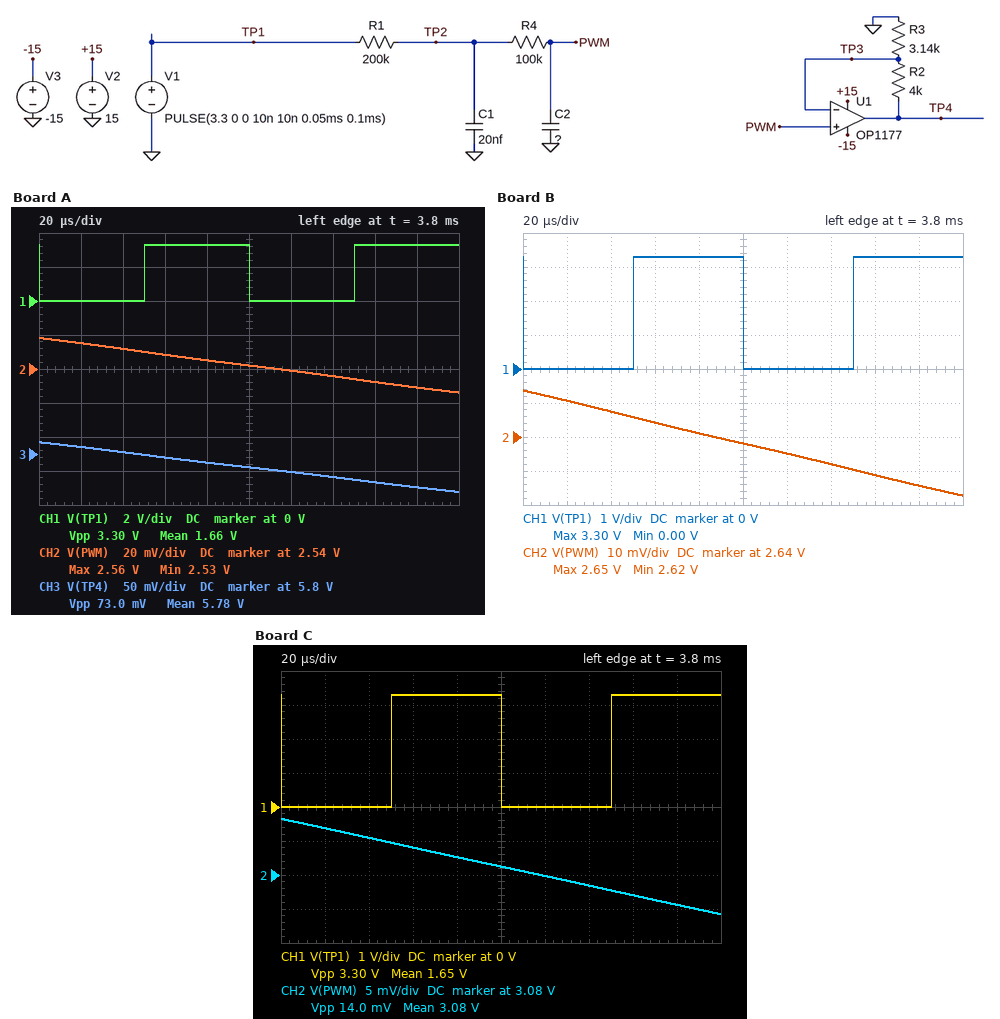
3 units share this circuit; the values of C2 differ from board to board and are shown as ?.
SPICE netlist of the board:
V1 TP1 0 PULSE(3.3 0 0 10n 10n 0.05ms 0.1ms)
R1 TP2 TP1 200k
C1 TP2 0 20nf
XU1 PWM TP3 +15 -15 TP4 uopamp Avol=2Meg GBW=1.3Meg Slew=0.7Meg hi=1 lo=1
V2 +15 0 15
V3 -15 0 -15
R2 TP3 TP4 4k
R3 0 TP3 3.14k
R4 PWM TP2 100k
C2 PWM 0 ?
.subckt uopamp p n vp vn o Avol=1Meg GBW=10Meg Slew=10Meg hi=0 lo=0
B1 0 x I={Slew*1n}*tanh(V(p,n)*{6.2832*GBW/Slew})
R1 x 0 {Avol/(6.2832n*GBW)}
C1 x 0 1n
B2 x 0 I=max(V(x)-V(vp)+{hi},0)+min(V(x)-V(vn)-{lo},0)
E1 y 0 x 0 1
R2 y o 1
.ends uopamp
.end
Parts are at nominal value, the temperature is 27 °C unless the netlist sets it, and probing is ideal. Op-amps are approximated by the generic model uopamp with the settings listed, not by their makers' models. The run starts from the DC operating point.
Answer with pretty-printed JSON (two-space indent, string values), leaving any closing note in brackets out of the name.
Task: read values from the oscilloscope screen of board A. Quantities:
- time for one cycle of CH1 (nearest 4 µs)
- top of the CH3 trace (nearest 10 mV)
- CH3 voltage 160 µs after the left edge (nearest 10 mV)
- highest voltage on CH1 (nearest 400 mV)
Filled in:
{
  "time for one cycle of CH1": "100 µs",
  "top of the CH3 trace": "5.82 V",
  "CH3 voltage 160 µs after the left edge": "5.76 V",
  "highest voltage on CH1": "3.2 V"
}
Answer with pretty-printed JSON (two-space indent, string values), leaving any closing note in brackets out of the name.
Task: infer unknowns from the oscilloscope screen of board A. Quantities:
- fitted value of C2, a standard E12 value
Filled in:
{
  "fitted value of C2, a standard E12 value": "6.8 nF"
}
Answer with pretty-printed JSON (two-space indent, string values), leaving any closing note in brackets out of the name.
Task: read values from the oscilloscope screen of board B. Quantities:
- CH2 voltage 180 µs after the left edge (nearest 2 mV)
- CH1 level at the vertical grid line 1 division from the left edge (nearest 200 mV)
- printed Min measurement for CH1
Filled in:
{
  "CH2 voltage 180 µs after the left edge": "2.626 V",
  "CH1 level at the vertical grid line 1 division from the left edge": "0 V",
  "printed Min measurement for CH1": "0.00 V"
}
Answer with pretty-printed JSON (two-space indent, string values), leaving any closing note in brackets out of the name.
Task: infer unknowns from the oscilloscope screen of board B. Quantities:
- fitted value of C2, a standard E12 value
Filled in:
{
  "fitted value of C2, a standard E12 value": "10 nF"
}
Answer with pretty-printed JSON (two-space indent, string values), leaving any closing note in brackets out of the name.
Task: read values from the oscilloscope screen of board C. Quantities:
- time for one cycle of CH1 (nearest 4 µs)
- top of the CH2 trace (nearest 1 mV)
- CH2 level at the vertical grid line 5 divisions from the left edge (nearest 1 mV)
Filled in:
{
  "time for one cycle of CH1": "100 µs",
  "top of the CH2 trace": "3.088 V",
  "CH2 level at the vertical grid line 5 divisions from the left edge": "3.081 V"
}
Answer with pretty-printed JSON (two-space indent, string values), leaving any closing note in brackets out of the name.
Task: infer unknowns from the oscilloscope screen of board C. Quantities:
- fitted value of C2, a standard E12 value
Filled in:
{
  "fitted value of C2, a standard E12 value": "56 nF"
}
